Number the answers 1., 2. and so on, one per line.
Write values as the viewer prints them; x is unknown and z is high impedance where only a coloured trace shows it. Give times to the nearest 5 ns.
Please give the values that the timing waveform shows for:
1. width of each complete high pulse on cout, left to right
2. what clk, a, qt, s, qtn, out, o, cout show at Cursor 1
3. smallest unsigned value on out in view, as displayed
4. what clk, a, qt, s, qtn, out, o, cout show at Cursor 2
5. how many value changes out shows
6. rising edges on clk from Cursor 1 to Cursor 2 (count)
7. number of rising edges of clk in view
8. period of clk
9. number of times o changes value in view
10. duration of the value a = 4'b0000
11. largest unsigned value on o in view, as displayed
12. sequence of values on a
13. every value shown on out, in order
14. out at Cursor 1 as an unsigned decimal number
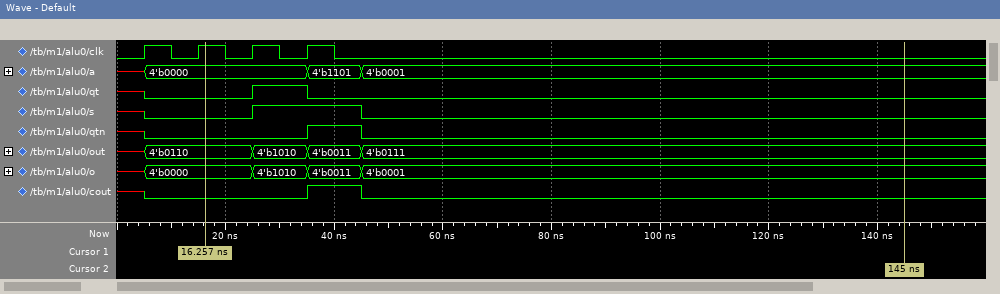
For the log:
1. 10 ns
2. clk=1, a=4'b0000, qt=0, s=0, qtn=0, out=4'b0110, o=4'b0000, cout=0
3. 4'b0011
4. clk=0, a=4'b0001, qt=0, s=0, qtn=0, out=4'b0111, o=4'b0001, cout=0
5. 4
6. 2
7. 4
8. 10 ns
9. 4
10. 30 ns
11. 4'b1010
12. x, 4'b0000, 4'b1101, 4'b0001
13. x, 4'b0110, 4'b1010, 4'b0011, 4'b0111
14. 6
